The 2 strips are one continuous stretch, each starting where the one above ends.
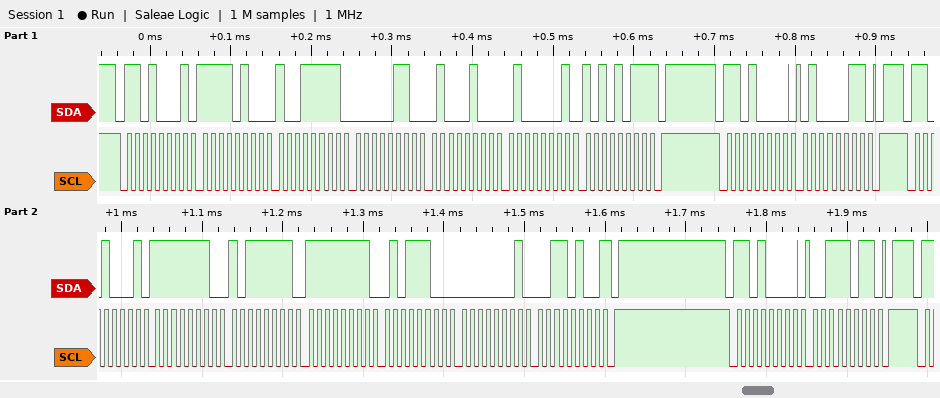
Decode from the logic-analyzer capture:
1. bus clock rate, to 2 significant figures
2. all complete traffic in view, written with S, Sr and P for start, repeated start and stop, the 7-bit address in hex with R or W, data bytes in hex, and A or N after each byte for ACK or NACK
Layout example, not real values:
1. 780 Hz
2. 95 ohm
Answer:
1. 100 kHz
2. S 68R A F4 A 9F A 06 A 44 A 41 A AB N P S 68W A 43 A P S 68R A FE A BF A FF A 5C A 01 A 34 N P S 68W A 3B A P
